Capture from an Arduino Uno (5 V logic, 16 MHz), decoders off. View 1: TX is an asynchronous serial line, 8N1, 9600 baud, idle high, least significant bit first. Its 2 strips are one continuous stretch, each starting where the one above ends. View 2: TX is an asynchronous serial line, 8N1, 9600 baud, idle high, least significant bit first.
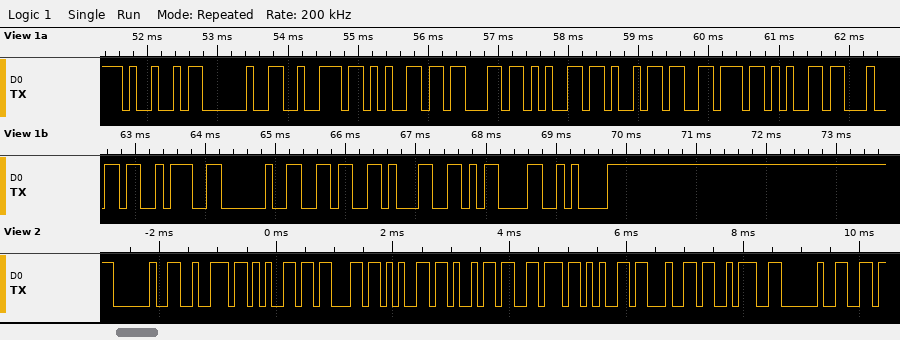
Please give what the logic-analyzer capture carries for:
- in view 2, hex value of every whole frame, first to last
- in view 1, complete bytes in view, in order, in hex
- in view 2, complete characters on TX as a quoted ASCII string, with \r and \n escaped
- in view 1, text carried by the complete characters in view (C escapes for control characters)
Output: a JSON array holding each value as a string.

["20 72 65 63 65 69 76 65 64 3A 20", "49 20 72 65 63 65 69 76 65 64 3A 20 36 31 0D 0A", "\" received: \"", "\"I received: 61\\r\\n\""]
